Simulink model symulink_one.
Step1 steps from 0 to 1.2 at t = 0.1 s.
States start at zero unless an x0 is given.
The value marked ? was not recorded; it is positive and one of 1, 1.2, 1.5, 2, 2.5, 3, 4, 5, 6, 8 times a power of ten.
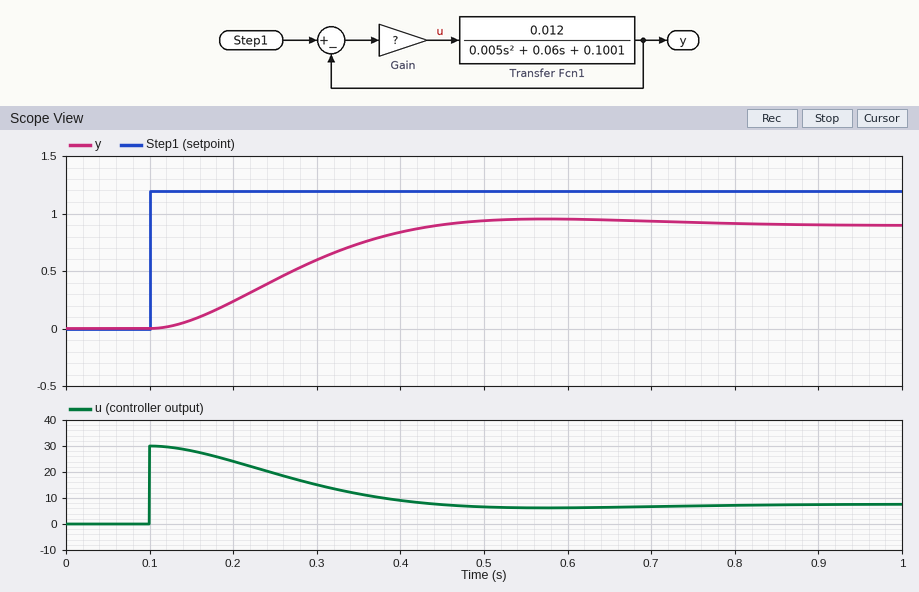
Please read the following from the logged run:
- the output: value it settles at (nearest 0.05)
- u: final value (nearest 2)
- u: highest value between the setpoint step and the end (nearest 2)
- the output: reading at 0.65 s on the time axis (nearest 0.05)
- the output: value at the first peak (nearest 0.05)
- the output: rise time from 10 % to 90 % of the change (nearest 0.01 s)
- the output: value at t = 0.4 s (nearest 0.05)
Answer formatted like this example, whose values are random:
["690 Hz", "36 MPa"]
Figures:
["0.90", "8", "30", "0.95", "0.95", "0.23 s", "0.85"]
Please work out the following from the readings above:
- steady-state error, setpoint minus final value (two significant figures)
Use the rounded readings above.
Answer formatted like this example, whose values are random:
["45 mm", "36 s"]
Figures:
["0.30"]
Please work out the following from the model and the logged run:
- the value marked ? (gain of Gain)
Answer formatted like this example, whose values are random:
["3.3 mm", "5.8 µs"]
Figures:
["25"]
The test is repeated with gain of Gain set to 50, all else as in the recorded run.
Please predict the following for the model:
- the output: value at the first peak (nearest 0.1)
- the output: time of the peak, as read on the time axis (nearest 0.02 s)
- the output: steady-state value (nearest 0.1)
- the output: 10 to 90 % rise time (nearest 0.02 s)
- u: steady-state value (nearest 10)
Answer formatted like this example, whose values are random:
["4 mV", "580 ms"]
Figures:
["1.2", "0.40 s", "1.0", "0.14 s", "10"]
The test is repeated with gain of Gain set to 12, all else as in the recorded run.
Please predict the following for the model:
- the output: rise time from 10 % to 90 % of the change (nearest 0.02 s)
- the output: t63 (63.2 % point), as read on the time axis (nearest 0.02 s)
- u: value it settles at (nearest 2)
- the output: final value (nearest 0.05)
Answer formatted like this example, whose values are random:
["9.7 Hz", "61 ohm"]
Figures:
["0.38 s", "0.38 s", "6", "0.70"]
